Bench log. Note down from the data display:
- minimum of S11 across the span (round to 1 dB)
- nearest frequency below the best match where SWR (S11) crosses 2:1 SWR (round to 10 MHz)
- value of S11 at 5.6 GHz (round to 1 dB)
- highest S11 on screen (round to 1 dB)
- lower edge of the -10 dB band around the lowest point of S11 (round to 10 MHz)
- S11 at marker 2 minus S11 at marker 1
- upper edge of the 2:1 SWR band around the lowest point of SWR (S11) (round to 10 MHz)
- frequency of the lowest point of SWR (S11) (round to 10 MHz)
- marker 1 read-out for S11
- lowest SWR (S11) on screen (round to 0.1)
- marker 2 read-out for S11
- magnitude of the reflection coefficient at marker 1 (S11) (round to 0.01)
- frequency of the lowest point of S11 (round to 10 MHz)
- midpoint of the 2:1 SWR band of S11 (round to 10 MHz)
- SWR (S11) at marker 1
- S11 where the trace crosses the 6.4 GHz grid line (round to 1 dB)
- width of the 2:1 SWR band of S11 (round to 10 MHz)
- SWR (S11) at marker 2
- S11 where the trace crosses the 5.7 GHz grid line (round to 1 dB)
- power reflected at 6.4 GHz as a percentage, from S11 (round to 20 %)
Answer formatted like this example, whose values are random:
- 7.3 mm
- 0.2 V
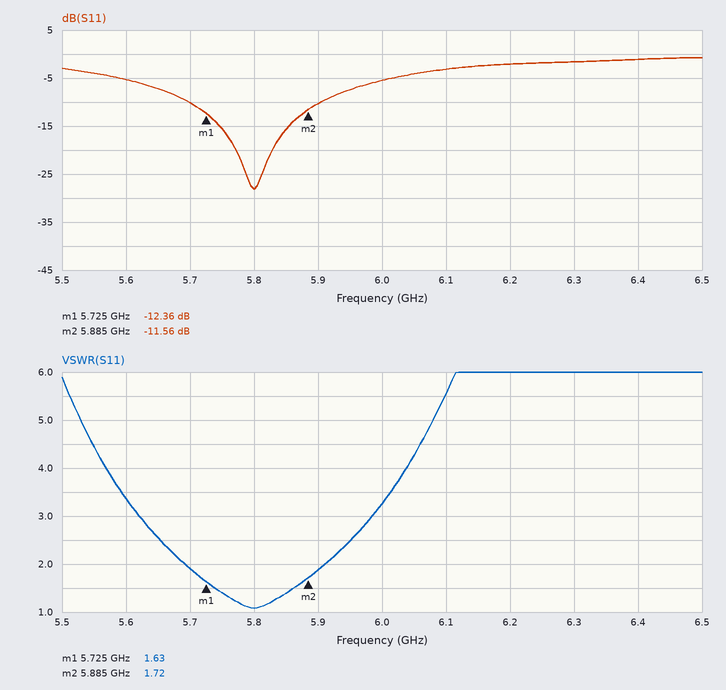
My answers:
- -28 dB
- 5.69 GHz
- -5 dB
- -1 dB
- 5.70 GHz
- 0.80 dB
- 5.91 GHz
- 5.80 GHz
- -12.36 dB
- 1.1
- -11.56 dB
- 0.24
- 5.80 GHz
- 5.80 GHz
- 1.63
- -1 dB
- 220 MHz
- 1.72
- -10 dB
- 80 %
